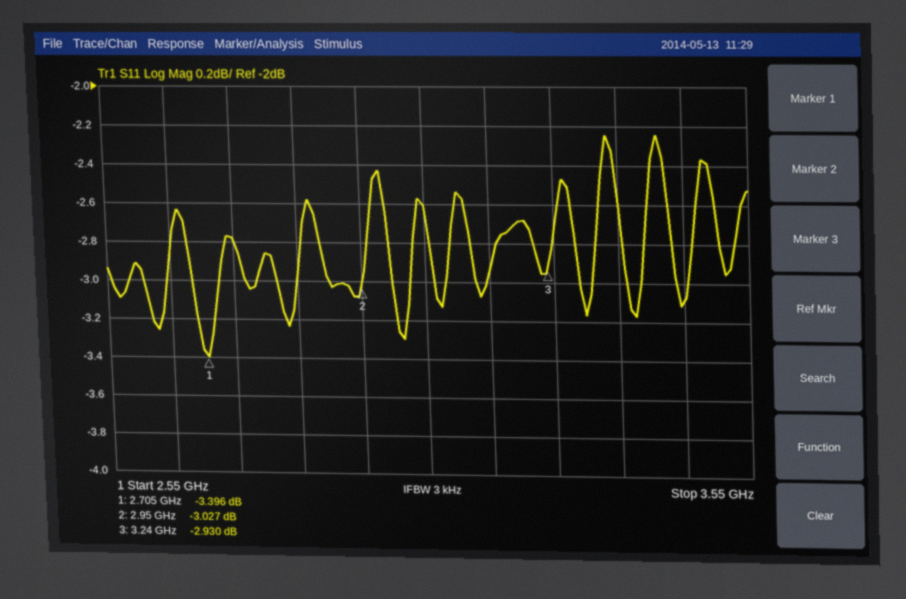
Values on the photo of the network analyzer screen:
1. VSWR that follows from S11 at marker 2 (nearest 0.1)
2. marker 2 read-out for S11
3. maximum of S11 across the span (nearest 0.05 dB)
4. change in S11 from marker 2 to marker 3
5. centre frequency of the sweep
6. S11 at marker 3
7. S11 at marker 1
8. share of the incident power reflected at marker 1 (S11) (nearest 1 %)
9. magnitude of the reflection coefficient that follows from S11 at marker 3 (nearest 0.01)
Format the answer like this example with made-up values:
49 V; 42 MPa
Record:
5.8; -3.027 dB; -2.25 dB; 0.097 dB; 3.05 GHz; -2.930 dB; -3.396 dB; 46 %; 0.71
